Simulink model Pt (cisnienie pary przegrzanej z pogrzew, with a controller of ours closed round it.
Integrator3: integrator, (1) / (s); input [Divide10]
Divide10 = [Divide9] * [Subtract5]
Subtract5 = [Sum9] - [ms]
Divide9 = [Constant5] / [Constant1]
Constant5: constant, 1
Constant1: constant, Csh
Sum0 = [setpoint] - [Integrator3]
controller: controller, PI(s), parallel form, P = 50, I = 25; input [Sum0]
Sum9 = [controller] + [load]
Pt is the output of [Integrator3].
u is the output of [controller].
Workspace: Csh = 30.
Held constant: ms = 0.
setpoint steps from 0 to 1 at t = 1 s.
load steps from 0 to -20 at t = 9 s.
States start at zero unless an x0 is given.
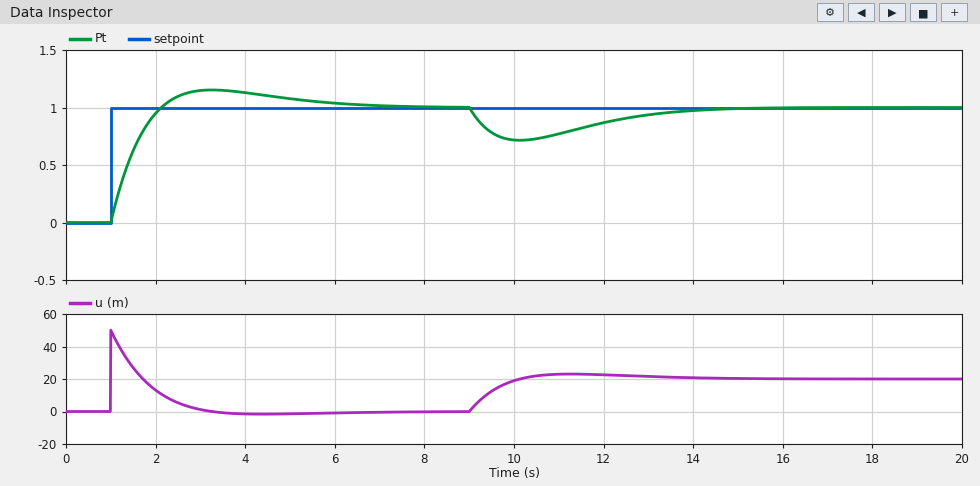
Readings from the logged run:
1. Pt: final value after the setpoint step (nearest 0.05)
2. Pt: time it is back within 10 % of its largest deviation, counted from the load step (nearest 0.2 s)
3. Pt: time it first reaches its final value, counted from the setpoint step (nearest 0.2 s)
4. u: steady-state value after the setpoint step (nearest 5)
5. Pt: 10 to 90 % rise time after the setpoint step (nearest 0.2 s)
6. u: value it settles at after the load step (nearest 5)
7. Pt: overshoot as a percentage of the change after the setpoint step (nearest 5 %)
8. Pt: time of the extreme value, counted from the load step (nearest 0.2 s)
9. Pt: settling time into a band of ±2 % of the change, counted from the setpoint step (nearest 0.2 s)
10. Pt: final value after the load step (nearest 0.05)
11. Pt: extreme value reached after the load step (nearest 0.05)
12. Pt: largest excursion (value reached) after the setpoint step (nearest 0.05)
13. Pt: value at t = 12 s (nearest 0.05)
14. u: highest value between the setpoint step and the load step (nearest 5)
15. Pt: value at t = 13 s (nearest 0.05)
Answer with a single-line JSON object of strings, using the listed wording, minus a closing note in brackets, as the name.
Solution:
{"Pt: final value after the setpoint step": "1.00", "Pt: time it is back within 10 % of its largest deviation, counted from the load step": "5.0 s", "Pt: time it first reaches its final value, counted from the setpoint step": "1.2 s", "u: steady-state value after the setpoint step": "0", "Pt: 10 to 90 % rise time after the setpoint step": "0.8 s", "u: value it settles at after the load step": "20", "Pt: overshoot as a percentage of the change after the setpoint step": "15 %", "Pt: time of the extreme value, counted from the load step": "1.2 s", "Pt: settling time into a band of ±2 % of the change, counted from the setpoint step": "5.8 s", "Pt: final value after the load step": "1.00", "Pt: extreme value reached after the load step": "0.70", "Pt: largest excursion (value reached) after the setpoint step": "1.15", "Pt: value at t = 12 s": "0.85", "u: highest value between the setpoint step and the load step": "50", "Pt: value at t = 13 s": "0.95"}
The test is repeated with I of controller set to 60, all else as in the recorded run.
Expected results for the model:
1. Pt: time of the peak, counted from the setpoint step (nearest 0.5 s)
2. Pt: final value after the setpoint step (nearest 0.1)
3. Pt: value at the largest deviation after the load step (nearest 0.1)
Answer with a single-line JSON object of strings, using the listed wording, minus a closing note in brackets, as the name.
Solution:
{"Pt: time of the peak, counted from the setpoint step": "1.5 s", "Pt: final value after the setpoint step": "1.0", "Pt: value at the largest deviation after the load step": "0.8"}
